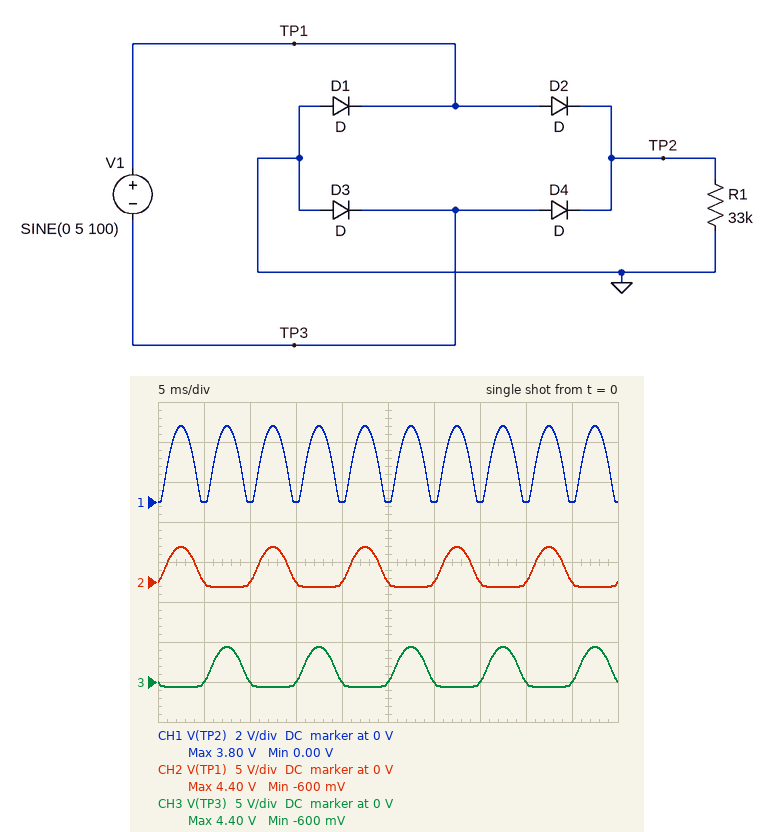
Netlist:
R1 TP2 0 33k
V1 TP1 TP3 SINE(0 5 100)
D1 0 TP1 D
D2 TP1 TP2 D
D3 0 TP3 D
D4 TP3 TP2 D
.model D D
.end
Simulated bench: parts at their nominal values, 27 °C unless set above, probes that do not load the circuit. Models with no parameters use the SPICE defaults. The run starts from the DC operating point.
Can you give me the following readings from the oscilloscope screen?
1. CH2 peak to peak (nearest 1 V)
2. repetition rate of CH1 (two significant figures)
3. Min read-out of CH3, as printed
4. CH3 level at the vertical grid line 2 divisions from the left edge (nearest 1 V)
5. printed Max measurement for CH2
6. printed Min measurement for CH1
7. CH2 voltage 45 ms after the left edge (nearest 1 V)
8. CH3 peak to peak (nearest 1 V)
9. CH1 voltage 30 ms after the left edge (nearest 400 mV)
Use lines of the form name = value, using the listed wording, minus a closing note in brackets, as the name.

CH2 peak to peak = 5 V
repetition rate of CH1 = 200 Hz
Min read-out of CH3, as printed = -600 mV
CH3 level at the vertical grid line 2 divisions from the left edge = 0 V
printed Max measurement for CH2 = 4.40 V
printed Min measurement for CH1 = 0.00 V
CH2 voltage 45 ms after the left edge = 0 V
CH3 peak to peak = 5 V
CH1 voltage 30 ms after the left edge = 0 V
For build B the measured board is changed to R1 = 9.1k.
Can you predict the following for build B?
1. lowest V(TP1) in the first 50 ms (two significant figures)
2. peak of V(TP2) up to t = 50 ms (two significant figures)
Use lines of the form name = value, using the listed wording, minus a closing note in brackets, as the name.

lowest V(TP1) in the first 50 ms = -630 mV
peak of V(TP2) up to t = 50 ms = 3.7 V
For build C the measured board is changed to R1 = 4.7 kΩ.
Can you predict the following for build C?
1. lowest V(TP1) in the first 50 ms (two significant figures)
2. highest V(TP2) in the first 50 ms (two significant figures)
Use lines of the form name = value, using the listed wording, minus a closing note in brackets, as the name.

lowest V(TP1) in the first 50 ms = -650 mV
highest V(TP2) in the first 50 ms = 3.7 V
